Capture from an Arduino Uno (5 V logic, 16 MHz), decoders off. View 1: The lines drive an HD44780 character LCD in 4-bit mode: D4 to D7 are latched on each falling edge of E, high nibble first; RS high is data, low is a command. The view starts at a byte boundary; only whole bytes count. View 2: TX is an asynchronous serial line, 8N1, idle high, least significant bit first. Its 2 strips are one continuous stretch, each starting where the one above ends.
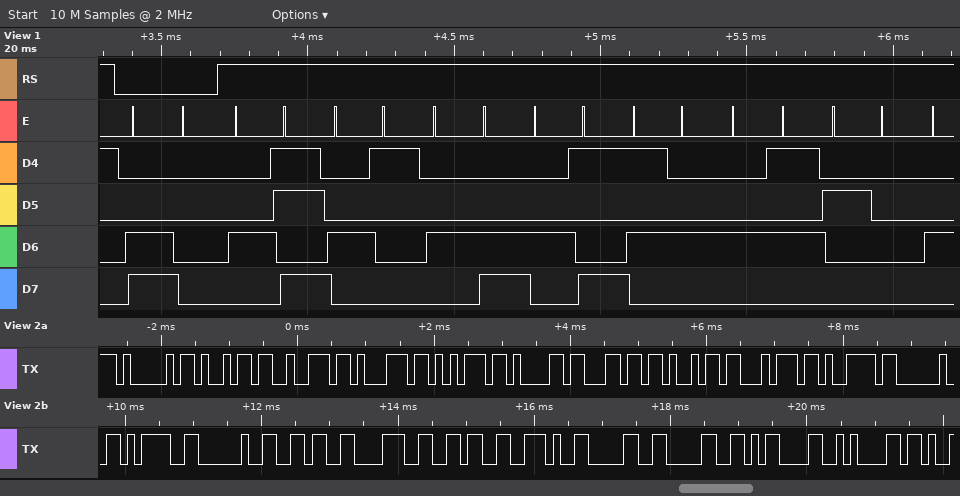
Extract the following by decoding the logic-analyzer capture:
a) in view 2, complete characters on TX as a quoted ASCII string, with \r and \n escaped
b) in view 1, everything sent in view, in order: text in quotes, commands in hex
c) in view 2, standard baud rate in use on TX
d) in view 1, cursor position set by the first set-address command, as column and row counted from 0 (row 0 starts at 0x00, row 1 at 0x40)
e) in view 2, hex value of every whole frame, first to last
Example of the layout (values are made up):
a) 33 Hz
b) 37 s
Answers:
a) "Airquality = 686.00\r\n"
b) 0xC0 "KALITE "
c) 9600 baud
d) column 0, row 1
e) 41 69 72 71 75 61 6C 69 74 79 20 3D 20 36 38 36 2E 30 30 0D 0A
